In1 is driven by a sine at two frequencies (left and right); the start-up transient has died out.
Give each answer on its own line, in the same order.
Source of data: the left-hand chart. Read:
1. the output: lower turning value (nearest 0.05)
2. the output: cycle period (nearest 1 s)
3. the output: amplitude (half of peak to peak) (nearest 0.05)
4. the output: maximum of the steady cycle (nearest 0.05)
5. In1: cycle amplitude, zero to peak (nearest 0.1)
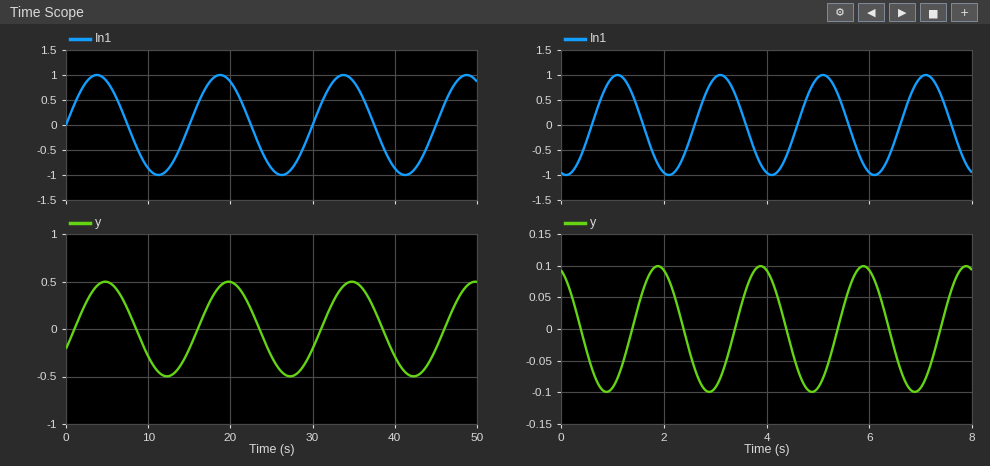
-0.50
15 s
0.50
0.50
1.0
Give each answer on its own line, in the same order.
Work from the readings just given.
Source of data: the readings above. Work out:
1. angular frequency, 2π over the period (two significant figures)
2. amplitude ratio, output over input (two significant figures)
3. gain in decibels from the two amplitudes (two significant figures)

0.42 rad/s
0.50
-6.0 dB
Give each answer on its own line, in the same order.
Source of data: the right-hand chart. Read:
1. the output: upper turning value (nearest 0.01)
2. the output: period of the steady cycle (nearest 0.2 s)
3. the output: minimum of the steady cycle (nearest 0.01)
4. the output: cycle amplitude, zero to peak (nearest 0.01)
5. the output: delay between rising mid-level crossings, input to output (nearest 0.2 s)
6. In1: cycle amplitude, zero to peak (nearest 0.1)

0.10
2.0 s
-0.10
0.10
0.8 s
1.0
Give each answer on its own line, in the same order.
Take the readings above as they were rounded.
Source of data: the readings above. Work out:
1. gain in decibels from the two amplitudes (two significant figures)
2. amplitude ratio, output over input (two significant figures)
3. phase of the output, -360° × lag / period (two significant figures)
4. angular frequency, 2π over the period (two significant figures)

-20 dB
0.10
-140°
3.1 rad/s
